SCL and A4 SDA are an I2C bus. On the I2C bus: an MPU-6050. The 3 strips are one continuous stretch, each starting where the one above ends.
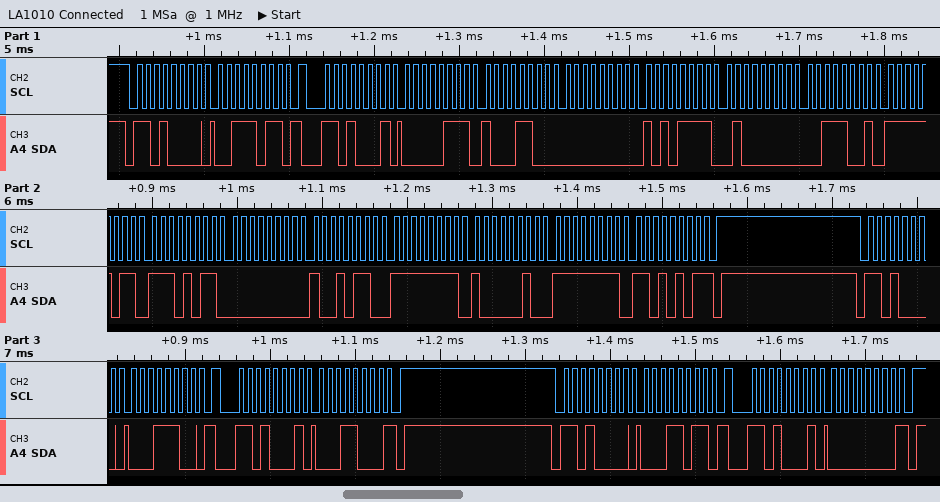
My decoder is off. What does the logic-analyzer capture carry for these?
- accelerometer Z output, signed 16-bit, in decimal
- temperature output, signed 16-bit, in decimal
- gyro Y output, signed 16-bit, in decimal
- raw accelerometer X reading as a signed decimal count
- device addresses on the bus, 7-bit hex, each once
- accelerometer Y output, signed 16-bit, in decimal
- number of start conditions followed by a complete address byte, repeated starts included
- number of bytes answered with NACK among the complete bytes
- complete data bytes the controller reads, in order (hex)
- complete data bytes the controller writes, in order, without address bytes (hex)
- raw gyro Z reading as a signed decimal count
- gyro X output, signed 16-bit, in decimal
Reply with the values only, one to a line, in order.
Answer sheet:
16441
-1045
-126
1932
0x68
175
6
3
07 8C 00 AF 40 39 FB EB 00 96 FF 82 FF D5 18 00
3B 1C 1B
-43
150
